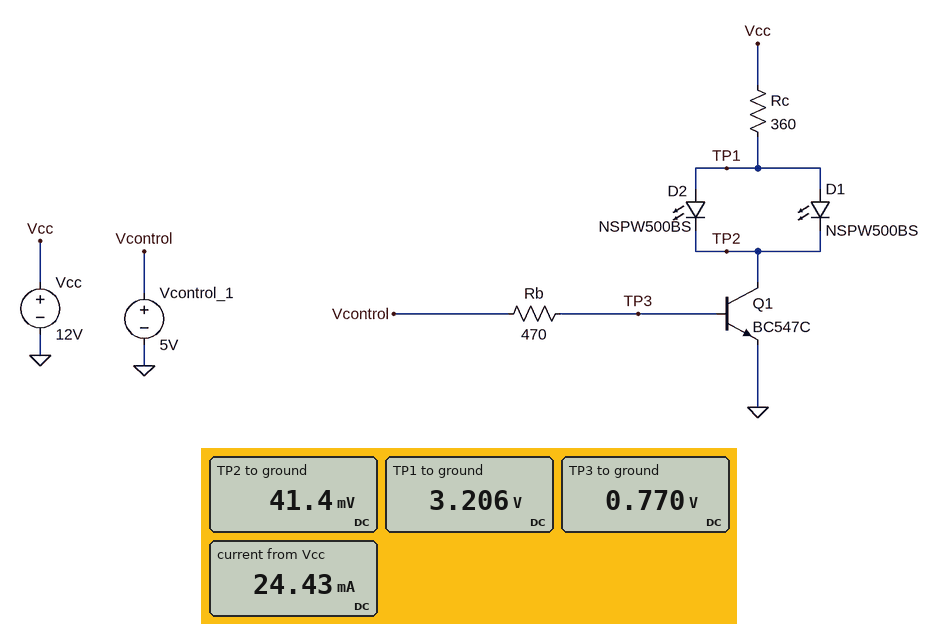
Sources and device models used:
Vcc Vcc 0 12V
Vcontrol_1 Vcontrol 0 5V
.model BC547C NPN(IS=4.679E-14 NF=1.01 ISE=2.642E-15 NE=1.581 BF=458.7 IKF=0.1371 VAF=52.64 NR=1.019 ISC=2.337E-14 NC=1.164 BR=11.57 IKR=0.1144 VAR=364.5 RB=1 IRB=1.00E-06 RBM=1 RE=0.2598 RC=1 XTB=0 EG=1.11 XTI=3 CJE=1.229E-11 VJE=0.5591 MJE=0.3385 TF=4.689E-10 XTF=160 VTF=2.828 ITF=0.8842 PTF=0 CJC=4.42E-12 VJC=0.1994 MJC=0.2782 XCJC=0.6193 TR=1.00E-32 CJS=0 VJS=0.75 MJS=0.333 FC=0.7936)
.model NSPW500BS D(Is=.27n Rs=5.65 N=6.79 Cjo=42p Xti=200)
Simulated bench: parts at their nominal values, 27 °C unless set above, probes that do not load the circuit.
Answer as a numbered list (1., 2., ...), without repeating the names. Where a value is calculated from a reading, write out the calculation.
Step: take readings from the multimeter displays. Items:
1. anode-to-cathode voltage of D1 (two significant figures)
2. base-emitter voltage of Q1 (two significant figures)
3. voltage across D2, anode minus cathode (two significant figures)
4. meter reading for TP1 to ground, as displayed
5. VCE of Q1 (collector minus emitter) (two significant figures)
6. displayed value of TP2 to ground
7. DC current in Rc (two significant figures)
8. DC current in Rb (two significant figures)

1. 3.206 V - 41.4 mV = 3.2 V
2. 770 mV = 770 mV
3. 3.206 V - 41.4 mV = 3.2 V
4. 3.206 V
5. 41.4 mV = 41 mV
6. 41.4 mV
7. (12 V - 3.206 V) / 360 Ω = 24 mA
8. (5 V - 770 mV) / 470 Ω = 9.0 mA
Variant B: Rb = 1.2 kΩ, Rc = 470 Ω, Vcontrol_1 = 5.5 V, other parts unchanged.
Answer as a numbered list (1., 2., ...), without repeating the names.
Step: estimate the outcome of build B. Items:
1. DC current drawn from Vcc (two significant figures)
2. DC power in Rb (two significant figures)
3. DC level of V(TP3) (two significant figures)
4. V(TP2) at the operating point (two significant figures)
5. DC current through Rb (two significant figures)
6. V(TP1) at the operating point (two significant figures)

1. 19 mA
2. 19 mW
3. 740 mV
4. 36 mV
5. 4.0 mA
6. 3.1 V
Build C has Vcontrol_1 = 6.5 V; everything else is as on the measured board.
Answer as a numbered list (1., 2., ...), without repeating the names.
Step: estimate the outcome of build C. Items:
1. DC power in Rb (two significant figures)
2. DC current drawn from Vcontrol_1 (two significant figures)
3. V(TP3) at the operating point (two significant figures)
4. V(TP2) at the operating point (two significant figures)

1. 70 mW
2. 12 mA
3. 780 mV
4. 41 mV
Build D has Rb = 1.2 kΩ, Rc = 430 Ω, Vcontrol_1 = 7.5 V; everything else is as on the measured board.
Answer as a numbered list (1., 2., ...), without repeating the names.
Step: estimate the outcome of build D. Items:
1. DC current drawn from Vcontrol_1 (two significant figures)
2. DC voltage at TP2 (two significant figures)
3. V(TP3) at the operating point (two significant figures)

1. 5.6 mA
2. 37 mV
3. 750 mV
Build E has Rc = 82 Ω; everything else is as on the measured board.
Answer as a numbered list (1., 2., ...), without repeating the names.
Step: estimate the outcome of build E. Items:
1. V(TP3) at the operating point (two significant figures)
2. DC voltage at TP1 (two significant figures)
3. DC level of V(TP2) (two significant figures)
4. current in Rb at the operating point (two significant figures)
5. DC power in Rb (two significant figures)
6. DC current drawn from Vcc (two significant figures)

1. 810 mV
2. 3.8 V
3. 160 mV
4. 8.9 mA
5. 37 mW
6. 100 mA
